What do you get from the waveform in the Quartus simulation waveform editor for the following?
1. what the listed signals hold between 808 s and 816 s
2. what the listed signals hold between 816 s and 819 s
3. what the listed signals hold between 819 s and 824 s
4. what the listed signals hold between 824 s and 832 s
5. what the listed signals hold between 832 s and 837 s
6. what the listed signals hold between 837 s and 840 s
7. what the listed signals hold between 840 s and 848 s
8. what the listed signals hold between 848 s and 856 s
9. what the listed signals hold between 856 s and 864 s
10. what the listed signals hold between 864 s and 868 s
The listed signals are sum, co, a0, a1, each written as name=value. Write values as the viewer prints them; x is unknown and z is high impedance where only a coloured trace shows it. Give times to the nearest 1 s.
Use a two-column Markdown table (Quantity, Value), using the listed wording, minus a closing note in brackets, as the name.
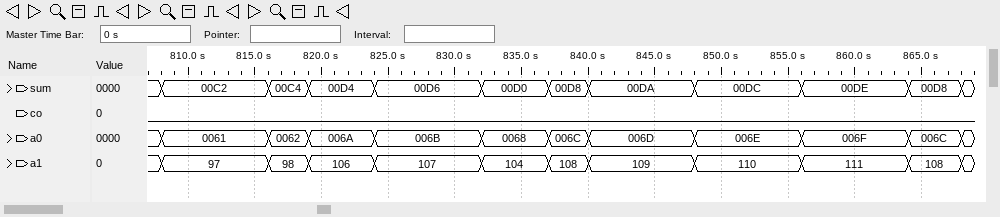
| Quantity | Value |
|---|---|
| what the listed signals hold between 808 s and 816 s | sum=00C2, co=0, a0=0061, a1=97 |
| what the listed signals hold between 816 s and 819 s | sum=00C4, co=0, a0=0062, a1=98 |
| what the listed signals hold between 819 s and 824 s | sum=00D4, co=0, a0=006A, a1=106 |
| what the listed signals hold between 824 s and 832 s | sum=00D6, co=0, a0=006B, a1=107 |
| what the listed signals hold between 832 s and 837 s | sum=00D0, co=0, a0=0068, a1=104 |
| what the listed signals hold between 837 s and 840 s | sum=00D8, co=0, a0=006C, a1=108 |
| what the listed signals hold between 840 s and 848 s | sum=00DA, co=0, a0=006D, a1=109 |
| what the listed signals hold between 848 s and 856 s | sum=00DC, co=0, a0=006E, a1=110 |
| what the listed signals hold between 856 s and 864 s | sum=00DE, co=0, a0=006F, a1=111 |
| what the listed signals hold between 864 s and 868 s | sum=00D8, co=0, a0=006C, a1=108 |
